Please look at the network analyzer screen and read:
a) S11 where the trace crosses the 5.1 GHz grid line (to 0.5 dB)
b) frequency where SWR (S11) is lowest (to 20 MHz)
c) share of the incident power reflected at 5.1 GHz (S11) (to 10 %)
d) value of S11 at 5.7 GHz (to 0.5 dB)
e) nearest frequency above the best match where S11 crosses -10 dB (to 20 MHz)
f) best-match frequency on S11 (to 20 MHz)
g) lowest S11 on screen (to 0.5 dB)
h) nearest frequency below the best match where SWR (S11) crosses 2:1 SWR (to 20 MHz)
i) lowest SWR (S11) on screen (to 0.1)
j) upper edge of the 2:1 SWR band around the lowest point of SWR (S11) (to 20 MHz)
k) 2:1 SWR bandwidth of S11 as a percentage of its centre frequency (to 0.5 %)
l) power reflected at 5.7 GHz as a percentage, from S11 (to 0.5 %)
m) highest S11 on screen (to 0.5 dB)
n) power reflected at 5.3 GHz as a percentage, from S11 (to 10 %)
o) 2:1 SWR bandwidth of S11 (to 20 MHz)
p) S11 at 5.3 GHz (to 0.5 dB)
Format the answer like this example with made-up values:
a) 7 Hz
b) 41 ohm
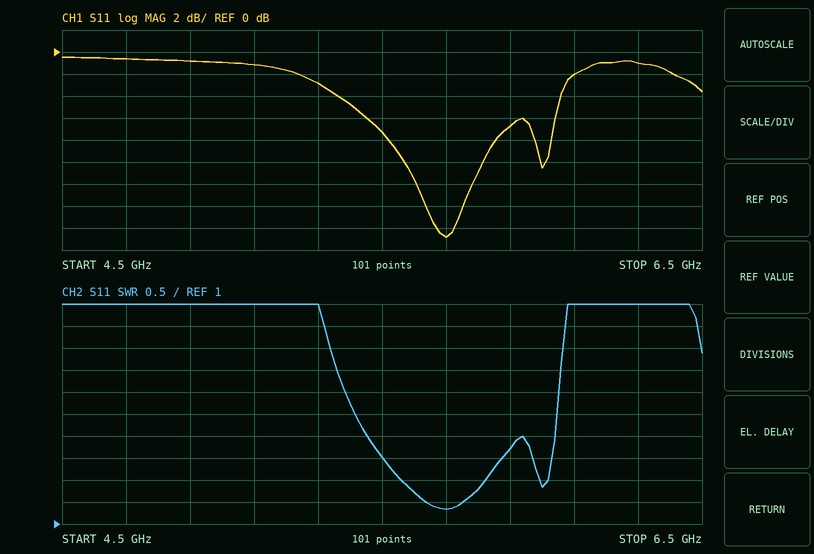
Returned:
a) -1.0 dB
b) 5.70 GHz
c) 80 %
d) -17.0 dB
e) 5.82 GHz
f) 5.70 GHz
g) -17.0 dB
h) 5.56 GHz
i) 1.3
j) 5.82 GHz
k) 4.5 %
l) 2.0 %
m) -0.5 dB
n) 50 %
o) 260 MHz
p) -3.0 dB
